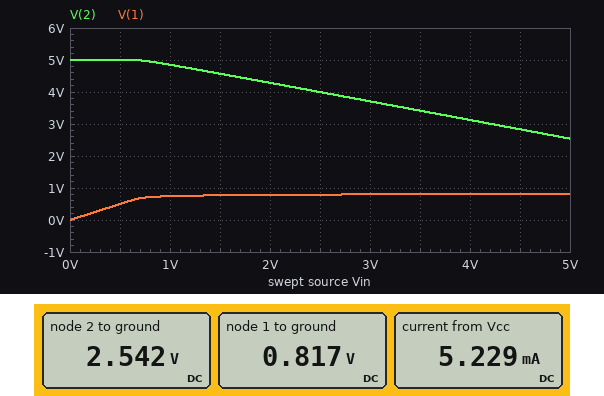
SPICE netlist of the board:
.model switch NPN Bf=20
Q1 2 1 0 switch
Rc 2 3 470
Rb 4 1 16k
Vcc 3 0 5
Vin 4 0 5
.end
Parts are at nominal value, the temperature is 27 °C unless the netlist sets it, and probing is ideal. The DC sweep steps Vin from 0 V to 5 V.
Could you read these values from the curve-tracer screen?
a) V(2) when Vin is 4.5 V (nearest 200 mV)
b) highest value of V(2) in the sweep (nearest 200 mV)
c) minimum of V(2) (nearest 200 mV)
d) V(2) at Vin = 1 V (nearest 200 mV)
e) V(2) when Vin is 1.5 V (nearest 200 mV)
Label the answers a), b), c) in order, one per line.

a) 2.8 V
b) 5.0 V
c) 2.6 V
d) 4.8 V
e) 4.6 V
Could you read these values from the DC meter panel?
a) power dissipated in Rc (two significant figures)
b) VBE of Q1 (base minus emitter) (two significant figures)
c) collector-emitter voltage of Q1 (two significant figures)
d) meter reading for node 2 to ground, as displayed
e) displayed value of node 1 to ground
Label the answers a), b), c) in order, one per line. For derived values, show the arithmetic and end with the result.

a) (5 V - 2.542 V)^2 / 470 Ω = 13 mW
b) 817 mV = 820 mV
c) 2.542 V = 2.5 V
d) 2.542 V
e) 0.817 V
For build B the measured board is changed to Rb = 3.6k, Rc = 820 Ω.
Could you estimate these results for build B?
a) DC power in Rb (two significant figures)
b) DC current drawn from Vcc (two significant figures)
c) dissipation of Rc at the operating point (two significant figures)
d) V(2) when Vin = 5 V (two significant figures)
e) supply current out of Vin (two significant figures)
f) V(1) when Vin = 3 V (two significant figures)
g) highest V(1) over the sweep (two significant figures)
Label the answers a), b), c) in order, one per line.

a) 4.8 mW
b) 6.0 mA
c) 30 mW
d) 59 mV
e) 1.2 mA
f) 820 mV
g) 830 mV
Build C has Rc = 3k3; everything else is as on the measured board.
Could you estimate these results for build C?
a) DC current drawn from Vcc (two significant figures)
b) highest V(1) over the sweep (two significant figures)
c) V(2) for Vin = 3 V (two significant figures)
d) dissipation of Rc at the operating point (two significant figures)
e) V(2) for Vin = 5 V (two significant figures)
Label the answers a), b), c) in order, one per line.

a) 1.5 mA
b) 790 mV
c) 86 mV
d) 7.4 mW
e) 61 mV
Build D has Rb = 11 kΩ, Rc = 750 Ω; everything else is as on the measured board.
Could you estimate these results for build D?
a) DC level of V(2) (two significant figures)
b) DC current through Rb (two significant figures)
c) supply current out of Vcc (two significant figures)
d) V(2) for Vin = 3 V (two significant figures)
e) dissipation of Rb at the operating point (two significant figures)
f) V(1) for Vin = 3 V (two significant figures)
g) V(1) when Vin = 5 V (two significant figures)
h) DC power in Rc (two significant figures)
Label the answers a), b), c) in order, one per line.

a) 130 mV
b) 380 µA
c) 6.5 mA
d) 2.0 V
e) 1.6 mW
f) 810 mV
g) 820 mV
h) 32 mW
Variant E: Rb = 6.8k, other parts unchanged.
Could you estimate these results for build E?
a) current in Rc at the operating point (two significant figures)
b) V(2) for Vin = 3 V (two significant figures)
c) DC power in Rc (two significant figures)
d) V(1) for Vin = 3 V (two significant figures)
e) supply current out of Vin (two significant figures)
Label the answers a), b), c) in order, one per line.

a) 10 mA
b) 2.0 V
c) 51 mW
d) 820 mV
e) 610 µA
